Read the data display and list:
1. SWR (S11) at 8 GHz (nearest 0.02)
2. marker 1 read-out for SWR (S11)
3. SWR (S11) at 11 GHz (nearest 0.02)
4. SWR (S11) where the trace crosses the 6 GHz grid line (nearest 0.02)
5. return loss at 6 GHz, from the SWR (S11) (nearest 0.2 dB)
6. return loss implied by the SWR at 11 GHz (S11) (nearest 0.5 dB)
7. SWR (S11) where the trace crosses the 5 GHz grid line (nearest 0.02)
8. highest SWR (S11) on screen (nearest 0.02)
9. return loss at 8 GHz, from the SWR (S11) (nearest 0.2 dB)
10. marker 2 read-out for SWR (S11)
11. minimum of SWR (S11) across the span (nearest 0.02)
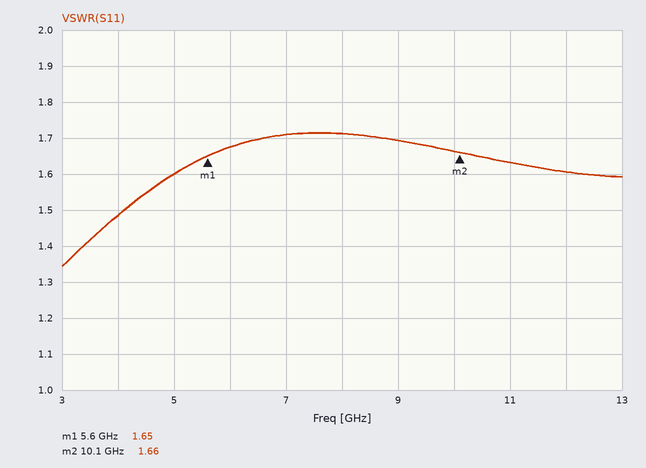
1.72
1.65
1.64
1.68
12.0 dB
12.5 dB
1.60
1.72
11.6 dB
1.66
1.34
